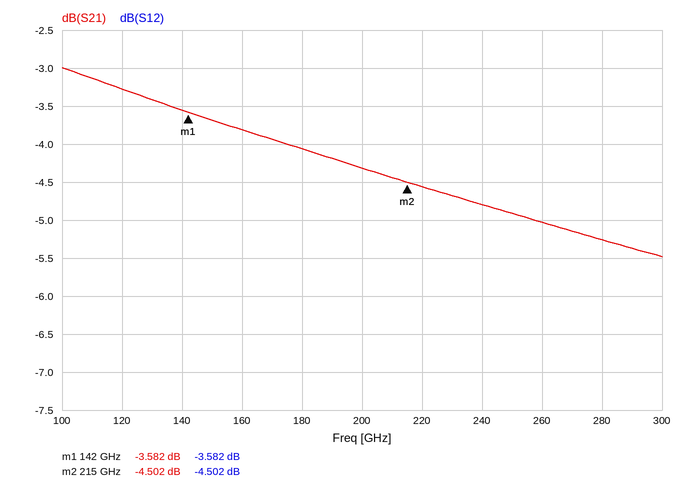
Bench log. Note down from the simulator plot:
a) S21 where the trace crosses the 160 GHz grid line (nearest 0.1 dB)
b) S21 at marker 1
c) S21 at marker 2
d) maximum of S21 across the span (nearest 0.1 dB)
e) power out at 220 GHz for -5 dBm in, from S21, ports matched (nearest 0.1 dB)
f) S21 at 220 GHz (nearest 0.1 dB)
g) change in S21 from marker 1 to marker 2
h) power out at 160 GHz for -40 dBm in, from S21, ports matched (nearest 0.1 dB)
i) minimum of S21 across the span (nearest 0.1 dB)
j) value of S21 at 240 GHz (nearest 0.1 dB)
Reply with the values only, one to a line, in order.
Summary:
-3.8 dB
-3.582 dB
-4.502 dB
-3.0 dB
-9.6 dBm
-4.6 dB
-0.920 dB
-43.8 dBm
-5.5 dB
-4.8 dB
